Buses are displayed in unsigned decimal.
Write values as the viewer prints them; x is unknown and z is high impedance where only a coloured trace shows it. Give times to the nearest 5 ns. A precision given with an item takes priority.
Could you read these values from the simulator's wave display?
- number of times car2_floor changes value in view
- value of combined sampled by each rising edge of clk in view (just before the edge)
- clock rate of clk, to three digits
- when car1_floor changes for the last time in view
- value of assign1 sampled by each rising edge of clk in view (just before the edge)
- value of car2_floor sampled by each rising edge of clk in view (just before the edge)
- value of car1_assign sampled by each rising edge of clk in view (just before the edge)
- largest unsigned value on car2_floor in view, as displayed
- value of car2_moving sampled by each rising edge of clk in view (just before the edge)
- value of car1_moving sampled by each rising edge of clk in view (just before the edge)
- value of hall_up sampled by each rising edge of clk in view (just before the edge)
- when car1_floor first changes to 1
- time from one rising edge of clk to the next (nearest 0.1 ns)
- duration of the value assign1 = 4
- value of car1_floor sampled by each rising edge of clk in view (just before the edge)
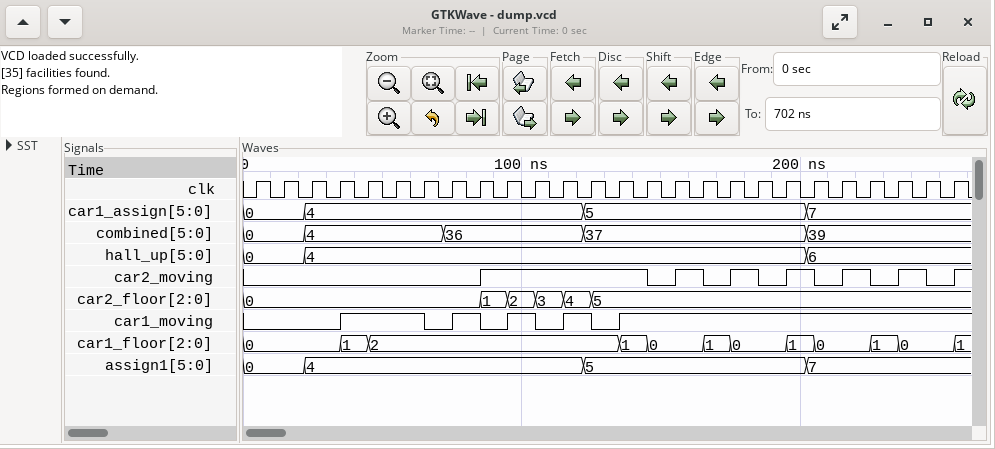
5
0, 0, 4, 4, 4, 4, 4, 36, 36, 36, 36, 36, 37, 37, 37, 37, 37, 37, 37, 37, 39, 39, 39, 39, 39, 39
100 MHz
255 ns
0, 0, 4, 4, 4, 4, 4, 4, 4, 4, 4, 4, 5, 5, 5, 5, 5, 5, 5, 5, 7, 7, 7, 7, 7, 7
0, 0, 0, 0, 0, 0, 0, 0, 0, 1, 2, 3, 4, 5, 5, 5, 5, 5, 5, 5, 5, 5, 5, 5, 5, 5
0, 0, 4, 4, 4, 4, 4, 4, 4, 4, 4, 4, 5, 5, 5, 5, 5, 5, 5, 5, 7, 7, 7, 7, 7, 7
5
0 0 0 0 0 0 0 0 0 1 1 1 1 1 1 0 1 0 1 0 1 0 1 0 1 0
0 0 0 0 1 1 1 0 1 0 1 0 1 0 1 1 1 1 1 1 1 1 1 1 1 1
0, 0, 4, 4, 4, 4, 4, 4, 4, 4, 4, 4, 4, 4, 4, 4, 4, 4, 4, 4, 6, 6, 6, 6, 6, 6
35 ns
10 ns
100 ns
0, 0, 0, 0, 1, 2, 2, 2, 2, 2, 2, 2, 2, 2, 1, 0, 0, 1, 0, 0, 1, 0, 0, 1, 0, 0
